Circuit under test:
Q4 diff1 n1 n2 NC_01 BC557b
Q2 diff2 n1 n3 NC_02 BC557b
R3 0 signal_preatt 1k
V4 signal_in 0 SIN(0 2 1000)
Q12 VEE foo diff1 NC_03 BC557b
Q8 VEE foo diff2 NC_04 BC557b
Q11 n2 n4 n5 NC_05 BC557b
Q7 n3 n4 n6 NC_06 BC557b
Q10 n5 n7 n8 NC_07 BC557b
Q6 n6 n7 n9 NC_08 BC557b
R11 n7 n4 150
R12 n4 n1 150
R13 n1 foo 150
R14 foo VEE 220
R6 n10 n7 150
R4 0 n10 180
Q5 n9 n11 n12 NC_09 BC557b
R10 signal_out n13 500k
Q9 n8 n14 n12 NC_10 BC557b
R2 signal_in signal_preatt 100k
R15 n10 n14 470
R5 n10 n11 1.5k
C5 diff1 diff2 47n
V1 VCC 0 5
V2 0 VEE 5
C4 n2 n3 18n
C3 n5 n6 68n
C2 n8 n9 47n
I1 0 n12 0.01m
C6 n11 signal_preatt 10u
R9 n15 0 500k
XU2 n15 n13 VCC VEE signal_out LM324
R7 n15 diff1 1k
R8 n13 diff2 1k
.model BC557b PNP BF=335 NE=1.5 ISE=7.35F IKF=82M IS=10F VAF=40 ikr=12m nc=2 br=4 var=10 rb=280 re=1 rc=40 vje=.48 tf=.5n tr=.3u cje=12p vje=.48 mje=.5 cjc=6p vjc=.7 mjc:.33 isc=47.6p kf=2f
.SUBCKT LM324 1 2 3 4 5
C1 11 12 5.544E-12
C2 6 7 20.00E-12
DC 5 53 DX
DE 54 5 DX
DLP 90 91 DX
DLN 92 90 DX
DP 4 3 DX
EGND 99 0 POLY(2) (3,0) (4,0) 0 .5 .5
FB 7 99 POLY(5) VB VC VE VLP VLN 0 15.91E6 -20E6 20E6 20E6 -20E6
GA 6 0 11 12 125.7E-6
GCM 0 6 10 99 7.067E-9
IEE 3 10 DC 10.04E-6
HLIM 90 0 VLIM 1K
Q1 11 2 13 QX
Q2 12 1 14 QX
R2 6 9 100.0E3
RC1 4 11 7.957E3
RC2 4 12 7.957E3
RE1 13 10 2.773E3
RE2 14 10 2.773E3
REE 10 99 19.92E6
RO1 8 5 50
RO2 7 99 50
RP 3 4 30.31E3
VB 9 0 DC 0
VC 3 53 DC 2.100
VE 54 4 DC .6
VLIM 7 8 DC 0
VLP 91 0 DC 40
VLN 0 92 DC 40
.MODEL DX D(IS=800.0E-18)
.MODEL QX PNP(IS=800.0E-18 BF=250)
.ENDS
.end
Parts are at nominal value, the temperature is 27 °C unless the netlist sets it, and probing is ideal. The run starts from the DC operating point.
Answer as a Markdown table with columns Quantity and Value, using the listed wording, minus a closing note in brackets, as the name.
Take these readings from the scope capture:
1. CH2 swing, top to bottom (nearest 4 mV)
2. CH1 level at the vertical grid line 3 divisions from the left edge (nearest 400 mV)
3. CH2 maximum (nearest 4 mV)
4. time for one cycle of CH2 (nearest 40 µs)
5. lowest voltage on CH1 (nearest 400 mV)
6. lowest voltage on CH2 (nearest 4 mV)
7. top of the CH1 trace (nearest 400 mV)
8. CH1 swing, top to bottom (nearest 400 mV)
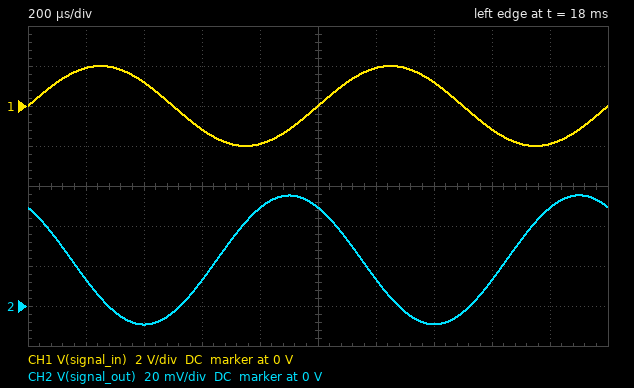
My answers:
| Quantity | Value |
|---|---|
| CH2 swing, top to bottom | 64 mV |
| CH1 level at the vertical grid line 3 divisions from the left edge | -1.2 V |
| CH2 maximum | 56 mV |
| time for one cycle of CH2 | 1.00 ms |
| lowest voltage on CH1 | -2.0 V |
| lowest voltage on CH2 | -8 mV |
| top of the CH1 trace | 2.0 V |
| CH1 swing, top to bottom | 4.0 V |
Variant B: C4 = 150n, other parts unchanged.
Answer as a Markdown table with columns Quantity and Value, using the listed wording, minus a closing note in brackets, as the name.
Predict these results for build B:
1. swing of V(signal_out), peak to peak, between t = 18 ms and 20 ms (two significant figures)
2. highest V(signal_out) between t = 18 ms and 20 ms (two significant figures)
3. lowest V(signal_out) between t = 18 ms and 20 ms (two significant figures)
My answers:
| Quantity | Value |
|---|---|
| swing of V(signal_out), peak to peak, between t = 18 ms and 20 ms | 10 mV |
| highest V(signal_out) between t = 18 ms and 20 ms | 28 mV |
| lowest V(signal_out) between t = 18 ms and 20 ms | 18 mV |
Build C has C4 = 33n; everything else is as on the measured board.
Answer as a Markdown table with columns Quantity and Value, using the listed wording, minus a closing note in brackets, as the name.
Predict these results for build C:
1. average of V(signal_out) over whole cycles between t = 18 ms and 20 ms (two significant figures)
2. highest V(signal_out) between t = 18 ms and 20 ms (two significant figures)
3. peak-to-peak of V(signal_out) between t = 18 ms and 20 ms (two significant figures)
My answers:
| Quantity | Value |
|---|---|
| average of V(signal_out) over whole cycles between t = 18 ms and 20 ms | 23 mV |
| highest V(signal_out) between t = 18 ms and 20 ms | 44 mV |
| peak-to-peak of V(signal_out) between t = 18 ms and 20 ms | 42 mV |
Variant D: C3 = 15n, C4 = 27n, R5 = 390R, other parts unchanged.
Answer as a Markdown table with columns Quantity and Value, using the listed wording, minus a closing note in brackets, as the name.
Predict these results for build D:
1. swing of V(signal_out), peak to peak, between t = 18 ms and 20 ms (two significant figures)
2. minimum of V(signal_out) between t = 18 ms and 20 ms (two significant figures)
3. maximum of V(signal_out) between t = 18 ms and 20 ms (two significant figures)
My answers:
| Quantity | Value |
|---|---|
| swing of V(signal_out), peak to peak, between t = 18 ms and 20 ms | 73 mV |
| minimum of V(signal_out) between t = 18 ms and 20 ms | -14 mV |
| maximum of V(signal_out) between t = 18 ms and 20 ms | 59 mV |
